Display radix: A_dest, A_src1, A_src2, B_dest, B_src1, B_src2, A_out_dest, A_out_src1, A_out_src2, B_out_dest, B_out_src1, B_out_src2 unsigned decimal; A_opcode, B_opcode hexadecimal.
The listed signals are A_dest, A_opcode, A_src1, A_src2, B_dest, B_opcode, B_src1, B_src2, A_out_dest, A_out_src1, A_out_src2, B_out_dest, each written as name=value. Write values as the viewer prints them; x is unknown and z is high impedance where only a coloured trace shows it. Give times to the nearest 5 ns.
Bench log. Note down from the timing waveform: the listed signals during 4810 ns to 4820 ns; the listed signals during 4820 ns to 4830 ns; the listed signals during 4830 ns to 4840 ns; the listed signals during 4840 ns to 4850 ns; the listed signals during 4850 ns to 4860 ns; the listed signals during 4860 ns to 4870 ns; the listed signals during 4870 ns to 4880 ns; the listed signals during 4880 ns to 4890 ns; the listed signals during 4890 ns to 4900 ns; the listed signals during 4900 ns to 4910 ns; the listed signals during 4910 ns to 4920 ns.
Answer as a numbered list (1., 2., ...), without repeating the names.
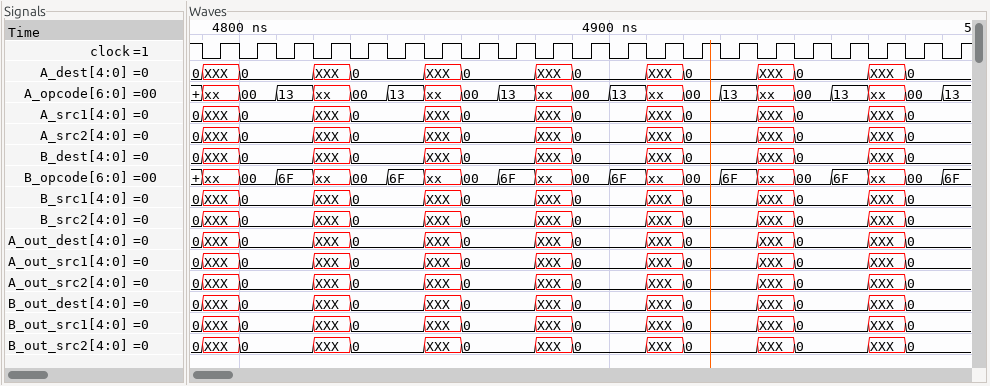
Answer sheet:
1. A_dest=0, A_opcode=13, A_src1=0, A_src2=0, B_dest=0, B_opcode=6F, B_src1=0, B_src2=0, A_out_dest=0, A_out_src1=0, A_out_src2=0, B_out_dest=0
2. A_dest=XXX, A_opcode=xx, A_src1=XXX, A_src2=XXX, B_dest=XXX, B_opcode=xx, B_src1=XXX, B_src2=XXX, A_out_dest=XXX, A_out_src1=XXX, A_out_src2=XXX, B_out_dest=XXX
3. A_dest=0, A_opcode=00, A_src1=0, A_src2=0, B_dest=0, B_opcode=00, B_src1=0, B_src2=0, A_out_dest=0, A_out_src1=0, A_out_src2=0, B_out_dest=0
4. A_dest=0, A_opcode=13, A_src1=0, A_src2=0, B_dest=0, B_opcode=6F, B_src1=0, B_src2=0, A_out_dest=0, A_out_src1=0, A_out_src2=0, B_out_dest=0
5. A_dest=XXX, A_opcode=xx, A_src1=XXX, A_src2=XXX, B_dest=XXX, B_opcode=xx, B_src1=XXX, B_src2=XXX, A_out_dest=XXX, A_out_src1=XXX, A_out_src2=XXX, B_out_dest=XXX
6. A_dest=0, A_opcode=00, A_src1=0, A_src2=0, B_dest=0, B_opcode=00, B_src1=0, B_src2=0, A_out_dest=0, A_out_src1=0, A_out_src2=0, B_out_dest=0
7. A_dest=0, A_opcode=13, A_src1=0, A_src2=0, B_dest=0, B_opcode=6F, B_src1=0, B_src2=0, A_out_dest=0, A_out_src1=0, A_out_src2=0, B_out_dest=0
8. A_dest=XXX, A_opcode=xx, A_src1=XXX, A_src2=XXX, B_dest=XXX, B_opcode=xx, B_src1=XXX, B_src2=XXX, A_out_dest=XXX, A_out_src1=XXX, A_out_src2=XXX, B_out_dest=XXX
9. A_dest=0, A_opcode=00, A_src1=0, A_src2=0, B_dest=0, B_opcode=00, B_src1=0, B_src2=0, A_out_dest=0, A_out_src1=0, A_out_src2=0, B_out_dest=0
10. A_dest=0, A_opcode=13, A_src1=0, A_src2=0, B_dest=0, B_opcode=6F, B_src1=0, B_src2=0, A_out_dest=0, A_out_src1=0, A_out_src2=0, B_out_dest=0
11. A_dest=XXX, A_opcode=xx, A_src1=XXX, A_src2=XXX, B_dest=XXX, B_opcode=xx, B_src1=XXX, B_src2=XXX, A_out_dest=XXX, A_out_src1=XXX, A_out_src2=XXX, B_out_dest=XXX
